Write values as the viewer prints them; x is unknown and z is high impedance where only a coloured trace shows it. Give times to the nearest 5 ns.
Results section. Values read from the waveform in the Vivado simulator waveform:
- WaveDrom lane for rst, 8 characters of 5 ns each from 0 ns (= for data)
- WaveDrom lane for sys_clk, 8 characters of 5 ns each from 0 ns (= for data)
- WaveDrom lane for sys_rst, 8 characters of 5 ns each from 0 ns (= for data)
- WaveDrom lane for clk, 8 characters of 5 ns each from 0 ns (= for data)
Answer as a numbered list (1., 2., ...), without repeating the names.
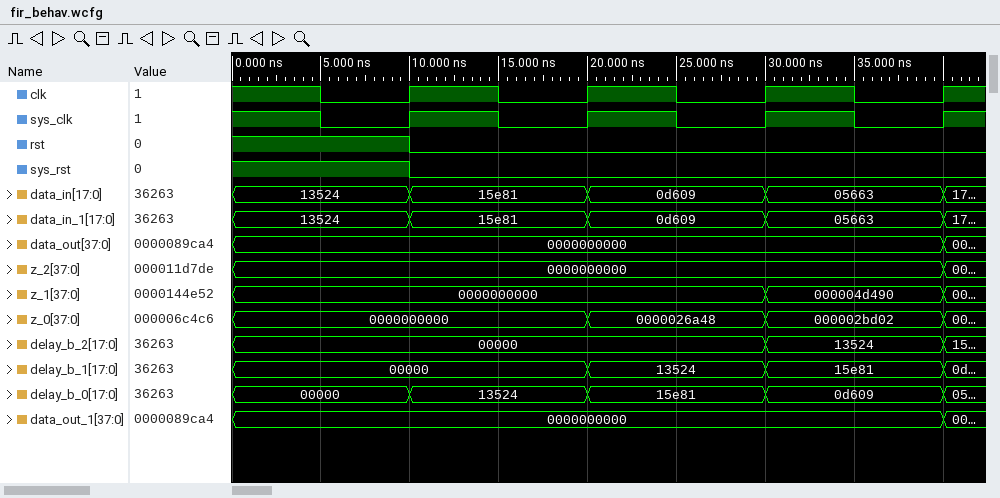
1. {name: 'rst', wave: '1.0.....'}
2. {name: 'sys_clk', wave: '10101010'}
3. {name: 'sys_rst', wave: '1.0.....'}
4. {name: 'clk', wave: '10101010'}
